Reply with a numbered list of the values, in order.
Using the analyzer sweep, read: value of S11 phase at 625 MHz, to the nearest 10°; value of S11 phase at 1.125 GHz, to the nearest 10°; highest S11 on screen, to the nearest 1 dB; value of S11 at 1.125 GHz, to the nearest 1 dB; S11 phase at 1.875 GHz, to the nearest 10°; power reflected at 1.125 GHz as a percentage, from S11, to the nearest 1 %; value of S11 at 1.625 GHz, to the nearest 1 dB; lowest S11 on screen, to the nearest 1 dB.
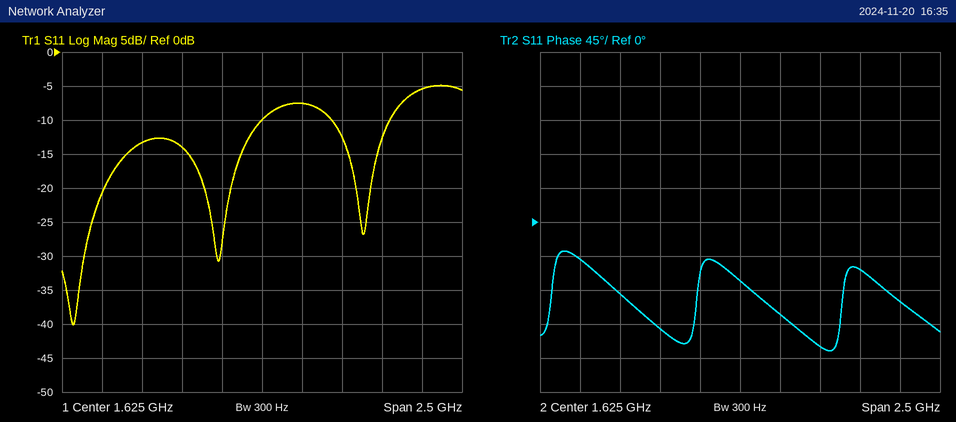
1. -50°
2. -140°
3. -5 dB
4. -14 dB
5. -120°
6. 4 %
7. -10 dB
8. -40 dB
